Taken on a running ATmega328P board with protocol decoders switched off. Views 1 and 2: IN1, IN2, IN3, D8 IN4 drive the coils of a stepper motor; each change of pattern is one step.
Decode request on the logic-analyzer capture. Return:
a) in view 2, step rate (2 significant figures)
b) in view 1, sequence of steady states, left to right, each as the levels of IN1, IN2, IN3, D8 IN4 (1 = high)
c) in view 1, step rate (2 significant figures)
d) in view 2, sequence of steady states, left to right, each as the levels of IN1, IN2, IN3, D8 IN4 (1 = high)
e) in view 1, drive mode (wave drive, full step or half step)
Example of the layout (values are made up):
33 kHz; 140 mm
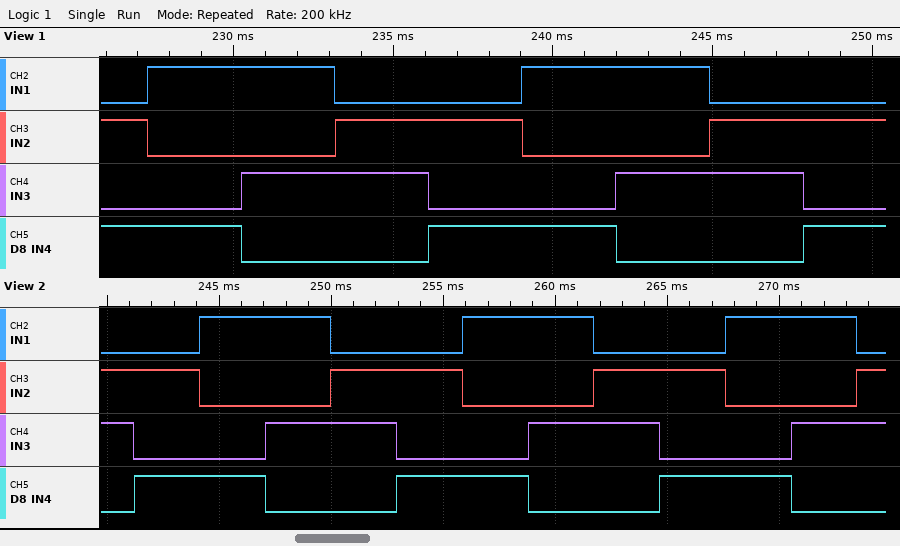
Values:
340 steps/s; 0101 1001 1010 0110 0101 1001 1010 0110 0101; 340 steps/s; 0110 0101 1001 1010 0110 0101 1001 1010 0110 0101 1001 1010 0110; full step
